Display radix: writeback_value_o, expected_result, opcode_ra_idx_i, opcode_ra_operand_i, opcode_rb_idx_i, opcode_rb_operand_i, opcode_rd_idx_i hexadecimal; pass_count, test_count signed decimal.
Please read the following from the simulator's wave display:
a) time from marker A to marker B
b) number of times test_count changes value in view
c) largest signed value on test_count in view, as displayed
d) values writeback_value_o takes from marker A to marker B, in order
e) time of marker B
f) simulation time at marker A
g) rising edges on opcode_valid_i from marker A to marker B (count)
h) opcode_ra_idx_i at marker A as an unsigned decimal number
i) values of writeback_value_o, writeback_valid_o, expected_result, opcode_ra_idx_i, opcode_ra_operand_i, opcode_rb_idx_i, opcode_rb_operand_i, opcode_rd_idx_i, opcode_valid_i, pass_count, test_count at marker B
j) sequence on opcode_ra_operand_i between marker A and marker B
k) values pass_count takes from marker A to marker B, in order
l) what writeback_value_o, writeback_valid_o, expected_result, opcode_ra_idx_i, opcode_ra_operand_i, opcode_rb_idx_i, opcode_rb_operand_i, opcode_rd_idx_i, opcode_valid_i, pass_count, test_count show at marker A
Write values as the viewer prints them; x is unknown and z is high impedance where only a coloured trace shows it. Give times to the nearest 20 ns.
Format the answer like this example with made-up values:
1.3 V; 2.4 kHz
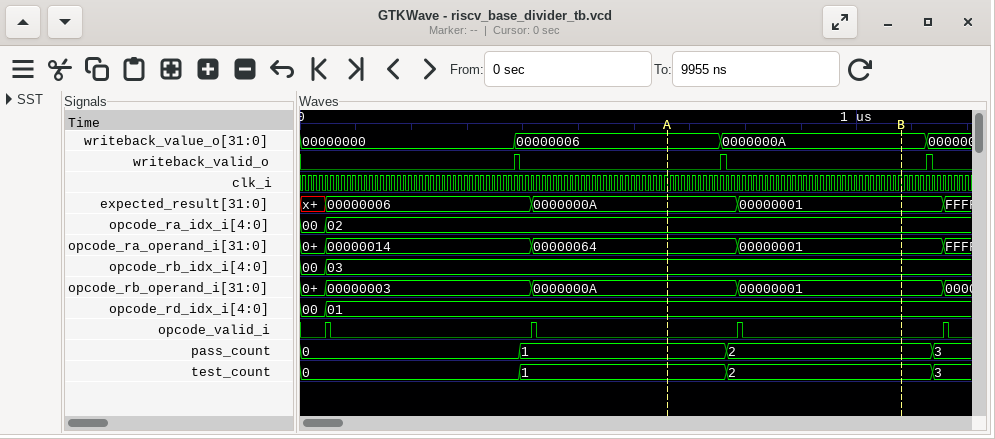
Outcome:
420 ns; 3; 3; 00000006, 0000000A; 1080 ns; 660 ns; 1; 2; writeback_value_o=0000000A, writeback_valid_o=0, expected_result=00000001, opcode_ra_idx_i=02, opcode_ra_operand_i=00000001, opcode_rb_idx_i=03, opcode_rb_operand_i=00000001, opcode_rd_idx_i=01, opcode_valid_i=0, pass_count=2, test_count=2; 00000064, 00000001; 1, 2; writeback_value_o=00000006, writeback_valid_o=0, expected_result=0000000A, opcode_ra_idx_i=02, opcode_ra_operand_i=00000064, opcode_rb_idx_i=03, opcode_rb_operand_i=0000000A, opcode_rd_idx_i=01, opcode_valid_i=0, pass_count=1, test_count=1
